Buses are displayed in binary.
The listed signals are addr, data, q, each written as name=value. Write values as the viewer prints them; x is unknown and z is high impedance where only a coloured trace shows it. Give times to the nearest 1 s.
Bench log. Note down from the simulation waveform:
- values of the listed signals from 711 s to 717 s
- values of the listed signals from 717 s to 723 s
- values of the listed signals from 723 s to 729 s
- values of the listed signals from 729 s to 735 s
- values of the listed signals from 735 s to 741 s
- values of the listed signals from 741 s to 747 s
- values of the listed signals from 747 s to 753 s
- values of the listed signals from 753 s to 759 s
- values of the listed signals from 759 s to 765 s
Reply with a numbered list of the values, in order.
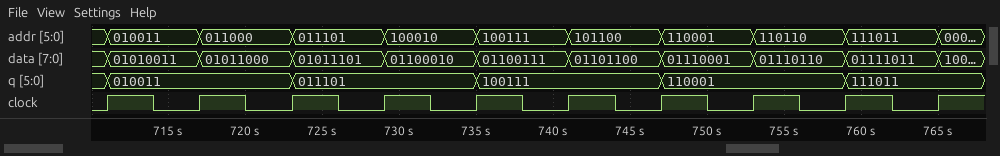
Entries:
1. addr=010011, data=01010011, q=010011
2. addr=011000, data=01011000, q=010011
3. addr=011101, data=01011101, q=011101
4. addr=100010, data=01100010, q=011101
5. addr=100111, data=01100111, q=100111
6. addr=101100, data=01101100, q=100111
7. addr=110001, data=01110001, q=110001
8. addr=110110, data=01110110, q=110001
9. addr=111011, data=01111011, q=111011
